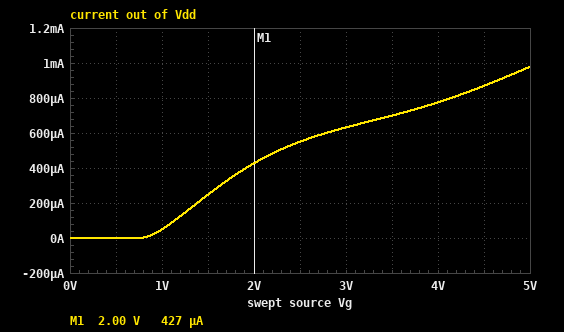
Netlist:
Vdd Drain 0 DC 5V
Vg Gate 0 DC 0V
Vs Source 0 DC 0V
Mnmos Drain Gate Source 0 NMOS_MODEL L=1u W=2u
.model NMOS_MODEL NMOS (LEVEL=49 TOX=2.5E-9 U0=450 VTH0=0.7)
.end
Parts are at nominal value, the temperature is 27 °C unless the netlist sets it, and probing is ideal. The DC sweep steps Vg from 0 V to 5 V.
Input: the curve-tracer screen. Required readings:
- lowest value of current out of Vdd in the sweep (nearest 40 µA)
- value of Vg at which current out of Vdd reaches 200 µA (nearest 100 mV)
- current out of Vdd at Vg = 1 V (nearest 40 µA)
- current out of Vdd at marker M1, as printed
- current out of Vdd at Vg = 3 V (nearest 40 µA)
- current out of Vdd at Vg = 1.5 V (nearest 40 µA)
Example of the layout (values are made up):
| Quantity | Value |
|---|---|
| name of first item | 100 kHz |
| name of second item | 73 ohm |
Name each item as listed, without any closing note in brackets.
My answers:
| Quantity | Value |
|---|---|
| lowest value of current out of Vdd in the sweep | 0 A |
| value of Vg at which current out of Vdd reaches 200 µA | 1.4 V |
| current out of Vdd at Vg = 1 V | 40 µA |
| current out of Vdd at marker M1, as printed | 427 µA |
| current out of Vdd at Vg = 3 V | 640 µA |
| current out of Vdd at Vg = 1.5 V | 240 µA |
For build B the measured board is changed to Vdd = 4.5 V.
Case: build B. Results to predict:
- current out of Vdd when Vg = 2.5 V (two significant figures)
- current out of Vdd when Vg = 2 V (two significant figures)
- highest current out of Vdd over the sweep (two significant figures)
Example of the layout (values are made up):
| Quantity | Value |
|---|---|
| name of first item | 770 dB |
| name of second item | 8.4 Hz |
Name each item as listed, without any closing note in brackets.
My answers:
| Quantity | Value |
|---|---|
| current out of Vdd when Vg = 2.5 V | 430 µA |
| current out of Vdd when Vg = 2 V | 320 µA |
| highest current out of Vdd over the sweep | 970 µA |
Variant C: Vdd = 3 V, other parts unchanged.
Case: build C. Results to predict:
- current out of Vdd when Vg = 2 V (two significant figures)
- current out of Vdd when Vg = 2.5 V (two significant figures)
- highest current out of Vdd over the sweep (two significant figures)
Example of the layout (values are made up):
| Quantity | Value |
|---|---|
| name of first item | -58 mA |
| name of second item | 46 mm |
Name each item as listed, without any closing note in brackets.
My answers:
| Quantity | Value |
|---|---|
| current out of Vdd when Vg = 2 V | 200 µA |
| current out of Vdd when Vg = 2.5 V | 330 µA |
| highest current out of Vdd over the sweep | 930 µA |
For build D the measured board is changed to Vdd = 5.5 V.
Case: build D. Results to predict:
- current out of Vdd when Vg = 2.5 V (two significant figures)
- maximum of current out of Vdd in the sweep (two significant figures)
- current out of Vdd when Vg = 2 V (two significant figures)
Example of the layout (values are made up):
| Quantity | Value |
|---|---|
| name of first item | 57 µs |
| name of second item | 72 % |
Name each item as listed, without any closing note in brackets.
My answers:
| Quantity | Value |
|---|---|
| current out of Vdd when Vg = 2.5 V | 740 µA |
| maximum of current out of Vdd in the sweep | 1.0 mA |
| current out of Vdd when Vg = 2 V | 580 µA |
